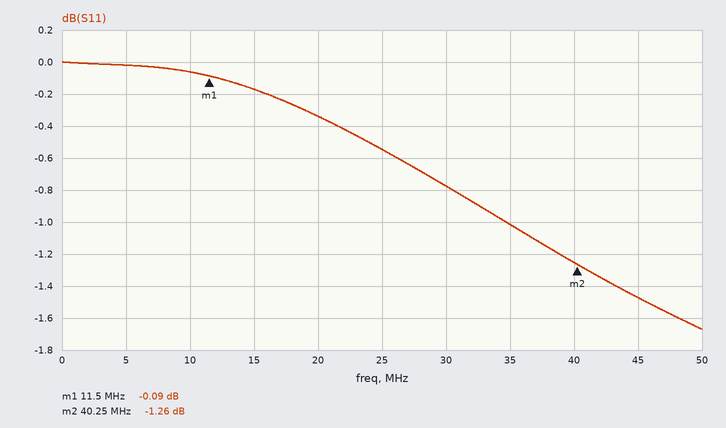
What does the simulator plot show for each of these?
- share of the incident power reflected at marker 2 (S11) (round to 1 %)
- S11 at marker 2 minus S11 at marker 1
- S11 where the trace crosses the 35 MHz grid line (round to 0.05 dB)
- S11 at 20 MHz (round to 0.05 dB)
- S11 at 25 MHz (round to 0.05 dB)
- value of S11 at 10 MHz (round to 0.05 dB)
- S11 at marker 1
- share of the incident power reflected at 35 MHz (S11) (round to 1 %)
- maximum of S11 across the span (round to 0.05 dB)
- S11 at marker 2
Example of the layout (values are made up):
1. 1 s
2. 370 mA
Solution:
1. 75 %
2. -1.17 dB
3. -1.00 dB
4. -0.35 dB
5. -0.55 dB
6. -0.05 dB
7. -0.09 dB
8. 79 %
9. 0.00 dB
10. -1.26 dB
